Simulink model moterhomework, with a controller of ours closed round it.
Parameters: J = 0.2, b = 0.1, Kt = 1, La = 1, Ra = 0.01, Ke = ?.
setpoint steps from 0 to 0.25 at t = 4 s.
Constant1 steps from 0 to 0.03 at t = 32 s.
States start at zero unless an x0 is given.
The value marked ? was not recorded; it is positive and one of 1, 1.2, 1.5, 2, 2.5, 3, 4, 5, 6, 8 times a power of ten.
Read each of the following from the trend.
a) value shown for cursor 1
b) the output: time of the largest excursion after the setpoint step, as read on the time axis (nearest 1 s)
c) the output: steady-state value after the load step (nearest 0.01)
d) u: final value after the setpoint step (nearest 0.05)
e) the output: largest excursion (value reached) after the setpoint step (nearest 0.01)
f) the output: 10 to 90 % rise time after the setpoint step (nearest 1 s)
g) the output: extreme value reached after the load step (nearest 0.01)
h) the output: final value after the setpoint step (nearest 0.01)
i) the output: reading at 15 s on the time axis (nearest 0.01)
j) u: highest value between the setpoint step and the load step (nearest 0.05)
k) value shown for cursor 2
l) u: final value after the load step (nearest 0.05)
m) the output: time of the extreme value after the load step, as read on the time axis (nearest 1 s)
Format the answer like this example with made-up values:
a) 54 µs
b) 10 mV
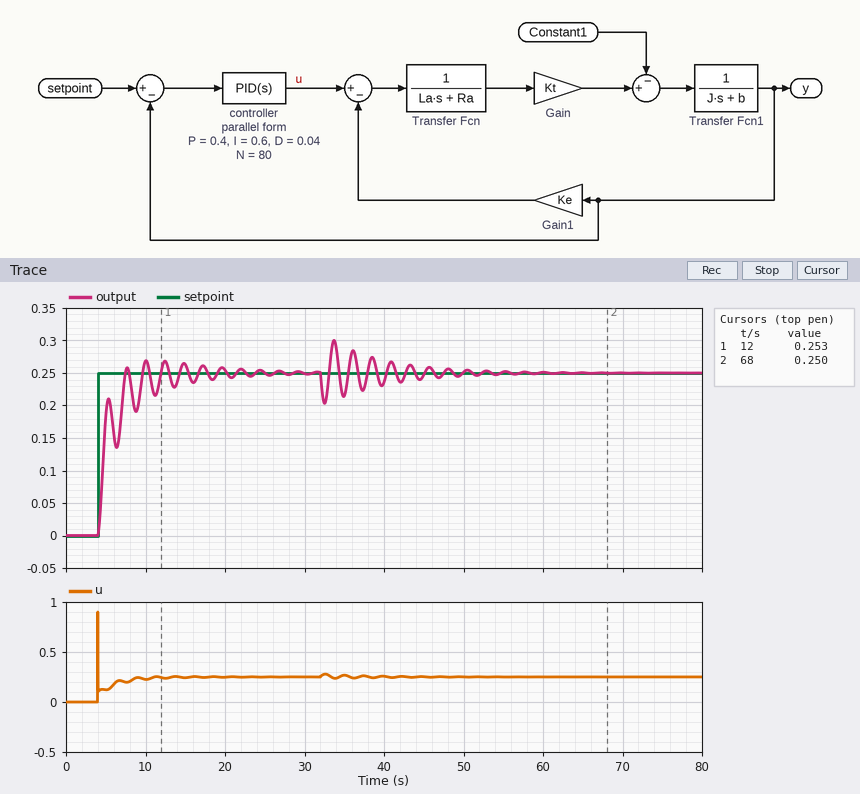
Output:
a) 0.253
b) 10 s
c) 0.25
d) 0.25
e) 0.27
f) 3 s
g) 0.30
h) 0.25
i) 0.26
j) 0.90
k) 0.250
l) 0.25
m) 34 s
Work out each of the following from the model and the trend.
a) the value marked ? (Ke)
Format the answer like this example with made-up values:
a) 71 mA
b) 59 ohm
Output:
a) 1
